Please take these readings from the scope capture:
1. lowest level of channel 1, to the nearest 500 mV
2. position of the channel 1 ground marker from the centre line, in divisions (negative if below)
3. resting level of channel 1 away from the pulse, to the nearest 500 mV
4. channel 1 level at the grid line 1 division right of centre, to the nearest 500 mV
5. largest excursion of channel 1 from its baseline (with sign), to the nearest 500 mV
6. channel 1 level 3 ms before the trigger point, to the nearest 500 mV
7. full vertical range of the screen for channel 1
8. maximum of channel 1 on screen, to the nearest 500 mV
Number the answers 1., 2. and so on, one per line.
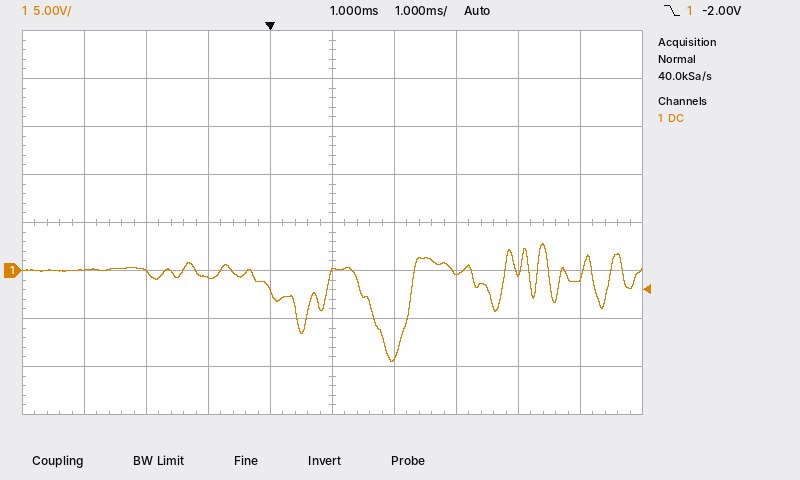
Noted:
1. -9.5 V
2. -1.0 div
3. 0.0 V
4. -9.0 V
5. -9.5 V
6. 0.0 V
7. 40 V
8. 3.0 V
